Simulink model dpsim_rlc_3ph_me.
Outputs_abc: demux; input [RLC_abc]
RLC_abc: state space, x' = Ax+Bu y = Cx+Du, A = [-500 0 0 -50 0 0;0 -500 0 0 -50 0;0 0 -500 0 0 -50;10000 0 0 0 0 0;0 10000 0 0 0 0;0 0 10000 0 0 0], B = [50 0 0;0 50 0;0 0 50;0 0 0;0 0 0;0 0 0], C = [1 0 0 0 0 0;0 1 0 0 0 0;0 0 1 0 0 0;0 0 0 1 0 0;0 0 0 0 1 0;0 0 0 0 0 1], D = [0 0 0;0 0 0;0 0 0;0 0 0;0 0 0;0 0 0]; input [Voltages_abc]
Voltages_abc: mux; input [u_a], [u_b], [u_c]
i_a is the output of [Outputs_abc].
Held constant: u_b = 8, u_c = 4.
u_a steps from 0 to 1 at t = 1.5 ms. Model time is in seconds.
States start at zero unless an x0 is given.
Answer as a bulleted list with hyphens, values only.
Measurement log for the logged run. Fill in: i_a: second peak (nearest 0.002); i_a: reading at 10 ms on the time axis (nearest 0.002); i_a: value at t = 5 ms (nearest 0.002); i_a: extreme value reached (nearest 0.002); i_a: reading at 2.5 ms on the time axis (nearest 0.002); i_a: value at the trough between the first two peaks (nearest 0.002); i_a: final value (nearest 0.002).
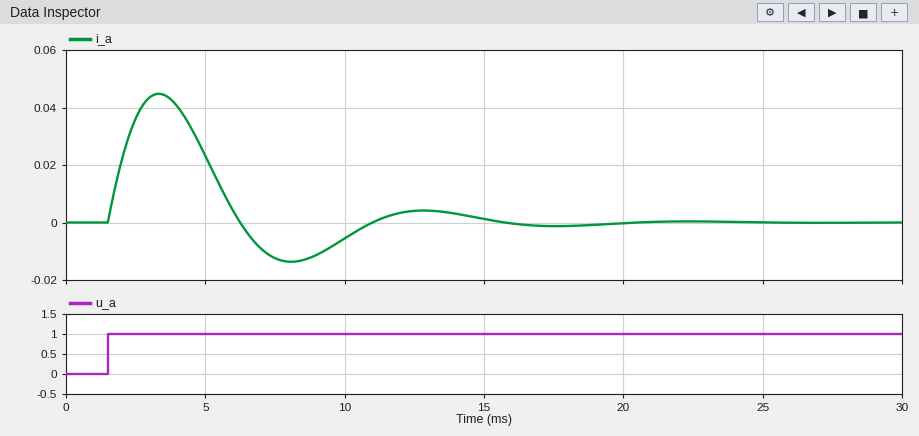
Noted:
- 0.004
- -0.006
- 0.024
- 0.044
- 0.036
- -0.014
- 0.000
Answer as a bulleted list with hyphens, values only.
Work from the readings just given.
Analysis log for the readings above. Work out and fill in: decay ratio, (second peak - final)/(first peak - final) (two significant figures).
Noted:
- 0.091
